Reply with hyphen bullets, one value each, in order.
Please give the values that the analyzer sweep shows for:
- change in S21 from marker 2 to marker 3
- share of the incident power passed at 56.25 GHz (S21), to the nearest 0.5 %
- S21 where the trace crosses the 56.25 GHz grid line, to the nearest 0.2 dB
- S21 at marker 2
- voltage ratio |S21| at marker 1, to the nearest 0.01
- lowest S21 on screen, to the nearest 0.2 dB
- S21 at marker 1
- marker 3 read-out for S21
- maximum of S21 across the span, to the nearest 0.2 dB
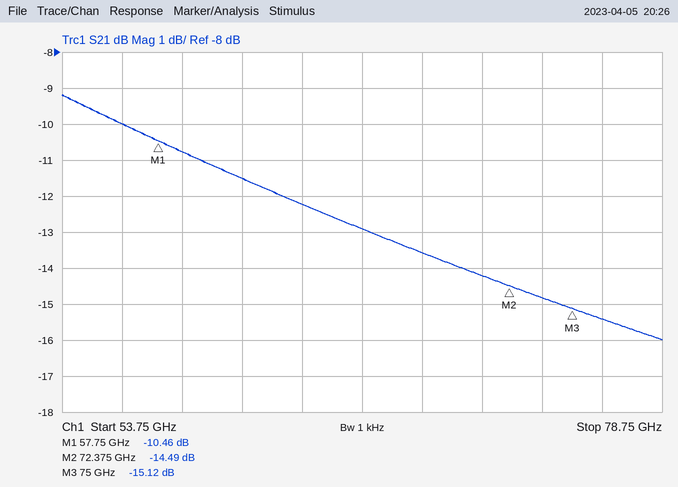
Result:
- -0.63 dB
- 10.0 %
- -10.0 dB
- -14.49 dB
- 0.30
- -16.0 dB
- -10.46 dB
- -15.12 dB
- -9.2 dB
